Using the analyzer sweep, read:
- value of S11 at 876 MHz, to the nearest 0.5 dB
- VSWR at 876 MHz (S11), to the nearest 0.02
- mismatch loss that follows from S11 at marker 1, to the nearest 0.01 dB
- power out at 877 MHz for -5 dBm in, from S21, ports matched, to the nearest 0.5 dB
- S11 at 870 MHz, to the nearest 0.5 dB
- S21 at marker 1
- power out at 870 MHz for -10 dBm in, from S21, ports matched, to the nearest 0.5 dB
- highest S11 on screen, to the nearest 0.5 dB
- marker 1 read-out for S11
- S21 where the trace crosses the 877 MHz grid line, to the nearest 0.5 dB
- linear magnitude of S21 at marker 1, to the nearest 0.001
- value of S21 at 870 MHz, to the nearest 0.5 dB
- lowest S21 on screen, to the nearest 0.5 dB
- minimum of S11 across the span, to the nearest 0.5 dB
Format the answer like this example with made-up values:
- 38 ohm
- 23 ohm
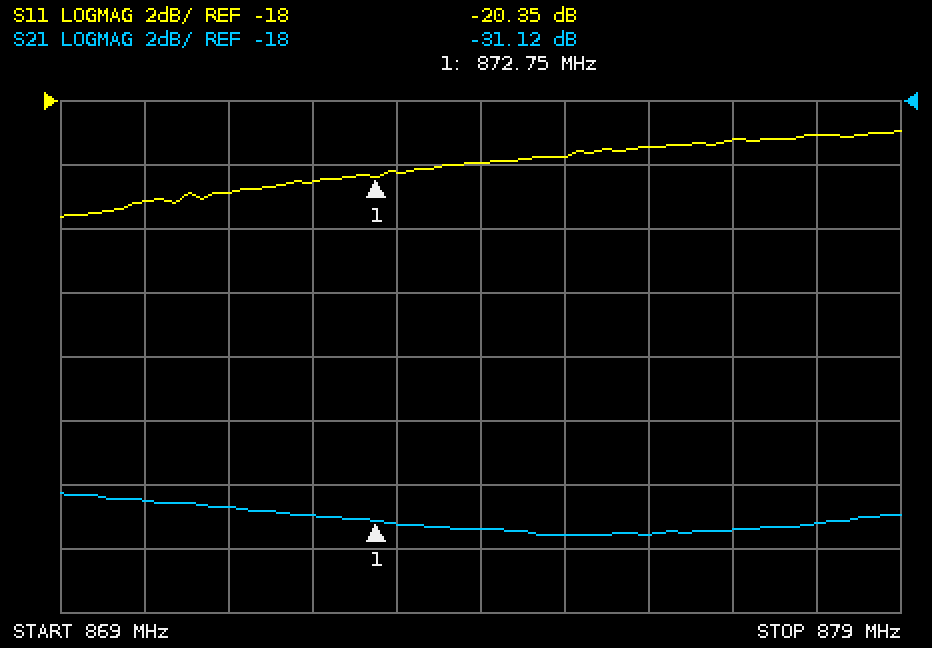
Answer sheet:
- -19.5 dB
- 1.24
- 0.04 dB
- -36.5 dBm
- -21.0 dB
- -31.12 dB
- -40.5 dBm
- -19.0 dB
- -20.35 dB
- -31.5 dB
- 0.028
- -30.5 dB
- -31.5 dB
- -21.5 dB
